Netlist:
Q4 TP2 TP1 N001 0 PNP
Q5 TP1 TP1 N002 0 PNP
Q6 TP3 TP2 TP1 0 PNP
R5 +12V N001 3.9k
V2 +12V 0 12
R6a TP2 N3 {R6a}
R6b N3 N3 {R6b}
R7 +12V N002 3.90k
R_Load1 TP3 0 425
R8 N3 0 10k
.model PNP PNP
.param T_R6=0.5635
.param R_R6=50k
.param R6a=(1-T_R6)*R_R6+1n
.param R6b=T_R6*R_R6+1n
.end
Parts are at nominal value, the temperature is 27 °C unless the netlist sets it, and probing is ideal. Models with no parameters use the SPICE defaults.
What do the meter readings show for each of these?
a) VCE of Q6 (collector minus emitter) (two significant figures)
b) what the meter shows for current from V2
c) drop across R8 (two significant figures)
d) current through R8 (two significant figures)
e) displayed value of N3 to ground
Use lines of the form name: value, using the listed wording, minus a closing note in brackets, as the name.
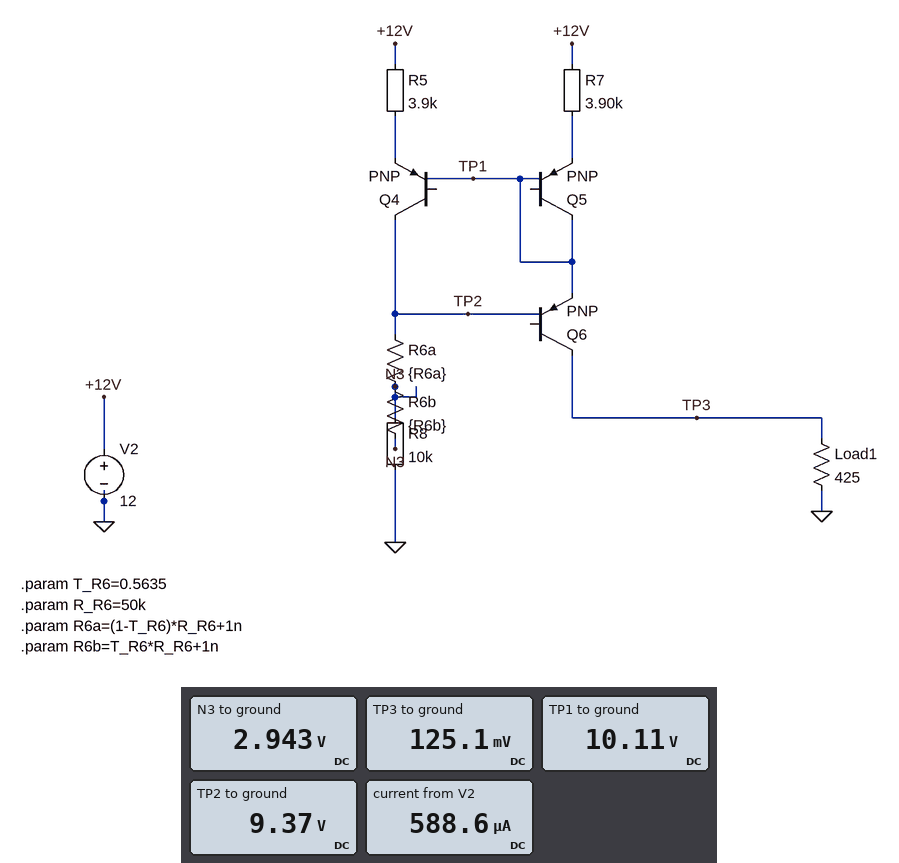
VCE of Q6 (collector minus emitter): -10 V
what the meter shows for current from V2: 588.6 µA
drop across R8: 2.9 V
current through R8: 290 µA
displayed value of N3 to ground: 2.943 V
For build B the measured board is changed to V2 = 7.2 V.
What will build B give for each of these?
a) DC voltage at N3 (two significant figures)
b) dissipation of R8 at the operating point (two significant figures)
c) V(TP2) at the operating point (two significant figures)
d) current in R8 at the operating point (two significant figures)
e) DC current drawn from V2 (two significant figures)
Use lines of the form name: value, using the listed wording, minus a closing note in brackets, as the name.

DC voltage at N3: 1.6 V
dissipation of R8 at the operating point: 260 µW
V(TP2) at the operating point: 5.1 V
current in R8 at the operating point: 160 µA
DC current drawn from V2: 320 µA
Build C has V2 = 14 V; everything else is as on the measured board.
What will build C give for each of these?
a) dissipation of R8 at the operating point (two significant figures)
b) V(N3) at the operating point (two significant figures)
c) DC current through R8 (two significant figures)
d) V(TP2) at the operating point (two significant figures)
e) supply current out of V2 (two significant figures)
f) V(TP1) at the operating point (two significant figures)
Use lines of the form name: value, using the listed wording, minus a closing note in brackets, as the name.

dissipation of R8 at the operating point: 1.2 mW
V(N3) at the operating point: 3.5 V
DC current through R8: 350 µA
V(TP2) at the operating point: 11 V
supply current out of V2: 700 µA
V(TP1) at the operating point: 12 V
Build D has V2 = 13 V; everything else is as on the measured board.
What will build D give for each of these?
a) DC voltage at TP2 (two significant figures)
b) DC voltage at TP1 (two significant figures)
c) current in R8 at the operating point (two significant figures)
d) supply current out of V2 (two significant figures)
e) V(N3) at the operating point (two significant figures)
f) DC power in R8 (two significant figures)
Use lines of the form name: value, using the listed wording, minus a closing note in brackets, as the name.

DC voltage at TP2: 10 V
DC voltage at TP1: 11 V
current in R8 at the operating point: 320 µA
supply current out of V2: 640 µA
V(N3) at the operating point: 3.2 V
DC power in R8: 1.0 mW
